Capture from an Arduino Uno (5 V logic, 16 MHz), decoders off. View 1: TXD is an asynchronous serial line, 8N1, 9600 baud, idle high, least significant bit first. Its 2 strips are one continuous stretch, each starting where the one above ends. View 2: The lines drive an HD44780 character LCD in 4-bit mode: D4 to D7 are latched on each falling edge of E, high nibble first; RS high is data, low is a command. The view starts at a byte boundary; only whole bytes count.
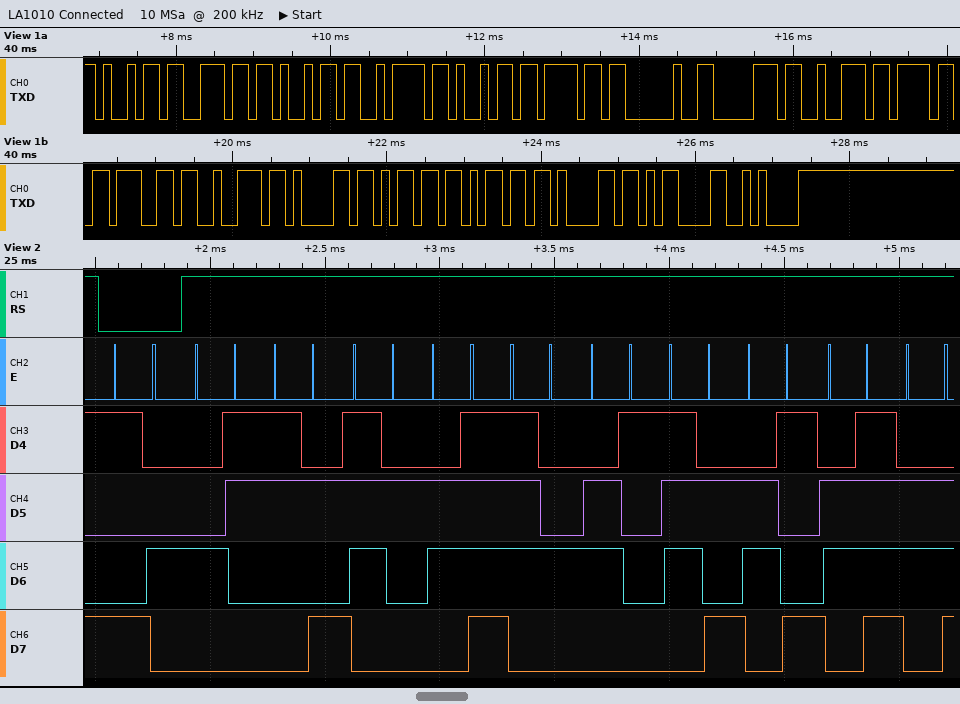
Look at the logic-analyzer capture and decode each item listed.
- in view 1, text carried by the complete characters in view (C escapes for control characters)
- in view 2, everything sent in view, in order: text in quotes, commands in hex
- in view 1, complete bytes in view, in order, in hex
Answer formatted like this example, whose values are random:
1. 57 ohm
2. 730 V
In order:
1. "inizio programma\r\n"
2. 0x94 "C:rotazion"
3. 0x69 0x6E 0x69 0x7A 0x69 0x6F 0x20 0x70 0x72 0x6F 0x67 0x72 0x61 0x6D 0x6D 0x61 0x0D 0x0A
